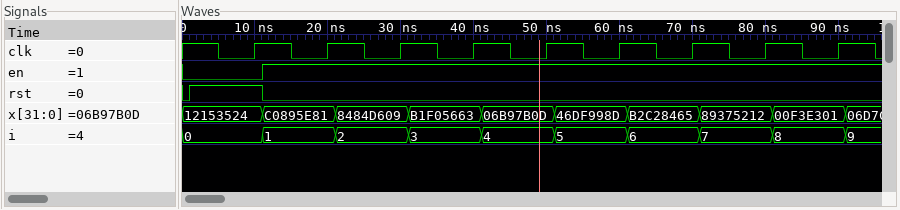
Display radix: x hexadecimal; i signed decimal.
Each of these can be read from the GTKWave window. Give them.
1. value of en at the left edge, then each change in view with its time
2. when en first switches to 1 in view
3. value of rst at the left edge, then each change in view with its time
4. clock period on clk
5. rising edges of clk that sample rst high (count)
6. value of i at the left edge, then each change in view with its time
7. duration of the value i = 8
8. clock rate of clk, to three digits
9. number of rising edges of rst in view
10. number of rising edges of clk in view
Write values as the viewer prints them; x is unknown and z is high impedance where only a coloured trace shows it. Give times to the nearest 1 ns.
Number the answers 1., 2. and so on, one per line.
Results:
1. 0, 1 at 11 ns
2. 11 ns
3. 0, 1 at 1 ns, 0 at 11 ns
4. 10 ns
5. 1
6. 0, 1 at 11 ns, 2 at 21 ns, 3 at 31 ns, 4 at 41 ns, 5 at 51 ns, 6 at 61 ns, 7 at 71 ns, 8 at 81 ns, 9 at 91 ns
7. 10 ns
8. 100 MHz
9. 1
10. 9
